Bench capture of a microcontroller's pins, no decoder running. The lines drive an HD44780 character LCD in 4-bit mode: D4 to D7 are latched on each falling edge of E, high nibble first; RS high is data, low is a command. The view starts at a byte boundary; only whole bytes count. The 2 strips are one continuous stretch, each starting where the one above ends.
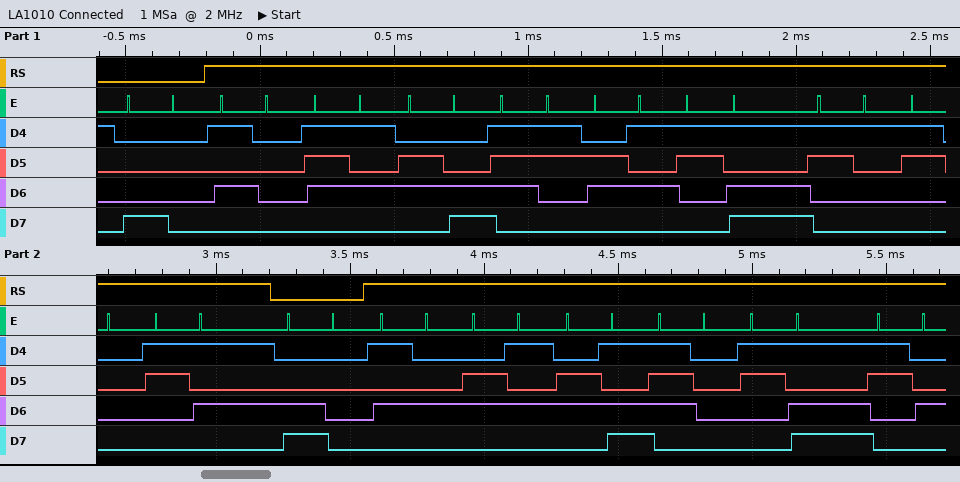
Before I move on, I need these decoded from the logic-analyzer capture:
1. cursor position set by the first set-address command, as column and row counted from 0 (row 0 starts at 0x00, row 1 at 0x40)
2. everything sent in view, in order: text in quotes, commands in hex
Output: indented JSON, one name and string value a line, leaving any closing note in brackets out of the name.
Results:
{
  "cursor position set by the first set-address command, as column and row counted from 0": "column 0, row 0",
  "everything sent in view, in order: text in quotes, commands in hex": "0x80 \"Pulse=105\" 0xC0 \"Temp=4\""
}
